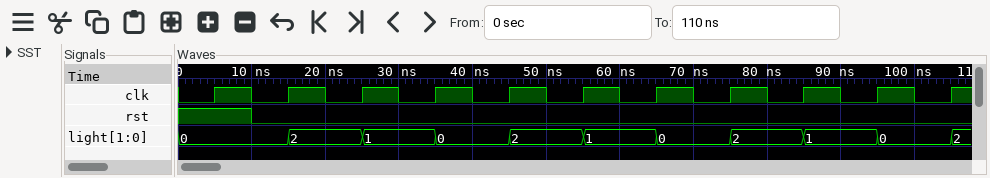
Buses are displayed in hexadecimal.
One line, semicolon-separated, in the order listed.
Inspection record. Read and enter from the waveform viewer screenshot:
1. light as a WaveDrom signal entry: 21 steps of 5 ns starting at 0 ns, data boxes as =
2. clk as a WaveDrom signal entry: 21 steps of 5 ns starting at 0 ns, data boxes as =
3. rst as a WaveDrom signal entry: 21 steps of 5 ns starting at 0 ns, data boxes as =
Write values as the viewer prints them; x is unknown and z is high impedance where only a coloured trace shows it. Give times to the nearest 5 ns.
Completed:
{name: 'light', wave: '=..=.=.=.=.=.=.=.=.=.', data: '0 2 1 0 2 1 0 2 1 0'}; {name: 'clk', wave: '010101010101010101010'}; {name: 'rst', wave: '1.0..................'}
